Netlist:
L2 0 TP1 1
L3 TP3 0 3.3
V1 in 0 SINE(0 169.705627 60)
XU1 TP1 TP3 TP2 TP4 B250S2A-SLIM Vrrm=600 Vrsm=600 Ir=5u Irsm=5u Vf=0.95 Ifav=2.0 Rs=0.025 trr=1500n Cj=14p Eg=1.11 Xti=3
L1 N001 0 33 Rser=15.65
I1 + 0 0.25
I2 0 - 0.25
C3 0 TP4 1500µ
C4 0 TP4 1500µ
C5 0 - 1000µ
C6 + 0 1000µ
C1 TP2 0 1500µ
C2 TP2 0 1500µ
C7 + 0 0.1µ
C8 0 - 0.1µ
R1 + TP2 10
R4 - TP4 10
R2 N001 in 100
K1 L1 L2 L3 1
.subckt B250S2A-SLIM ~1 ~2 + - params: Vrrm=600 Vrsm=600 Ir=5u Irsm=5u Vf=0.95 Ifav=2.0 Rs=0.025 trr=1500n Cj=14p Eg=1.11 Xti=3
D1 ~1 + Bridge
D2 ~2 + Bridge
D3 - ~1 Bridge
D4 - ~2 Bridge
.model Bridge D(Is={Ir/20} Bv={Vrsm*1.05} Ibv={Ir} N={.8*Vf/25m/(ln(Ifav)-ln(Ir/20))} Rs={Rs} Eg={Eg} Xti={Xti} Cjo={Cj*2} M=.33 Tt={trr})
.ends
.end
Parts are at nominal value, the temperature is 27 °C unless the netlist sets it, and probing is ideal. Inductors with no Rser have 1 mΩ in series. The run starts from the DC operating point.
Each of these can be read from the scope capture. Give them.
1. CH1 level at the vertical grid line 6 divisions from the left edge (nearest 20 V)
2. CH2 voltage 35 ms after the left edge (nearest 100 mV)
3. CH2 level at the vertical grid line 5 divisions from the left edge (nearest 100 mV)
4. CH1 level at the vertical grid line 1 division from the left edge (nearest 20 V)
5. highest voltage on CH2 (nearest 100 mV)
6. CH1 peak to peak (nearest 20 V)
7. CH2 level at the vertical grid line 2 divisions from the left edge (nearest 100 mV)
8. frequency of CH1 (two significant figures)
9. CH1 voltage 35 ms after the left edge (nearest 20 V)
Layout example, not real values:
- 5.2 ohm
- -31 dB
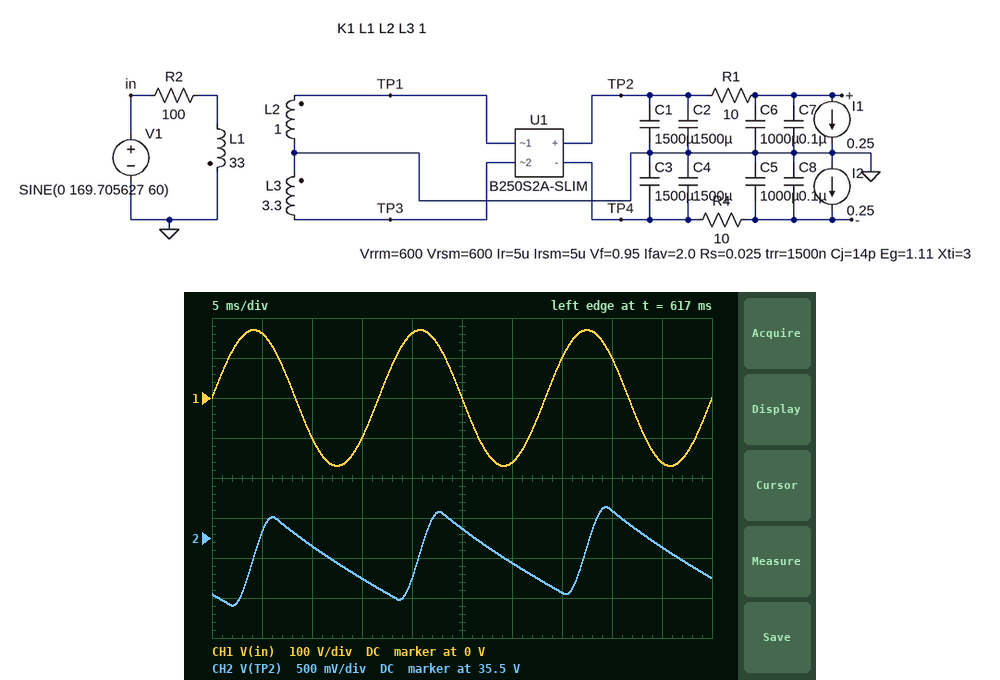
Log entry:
- -160 V
- 34.8 V
- 35.6 V
- 160 V
- 35.9 V
- 340 V
- 35.4 V
- 60 Hz
- 100 V
